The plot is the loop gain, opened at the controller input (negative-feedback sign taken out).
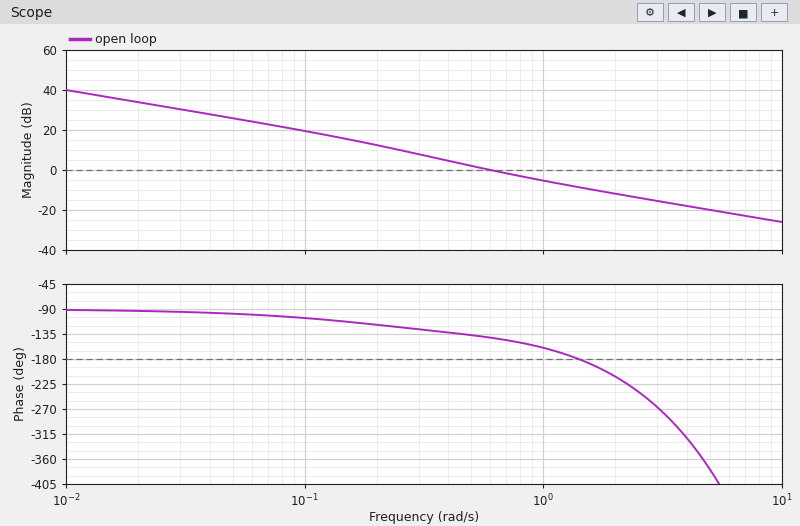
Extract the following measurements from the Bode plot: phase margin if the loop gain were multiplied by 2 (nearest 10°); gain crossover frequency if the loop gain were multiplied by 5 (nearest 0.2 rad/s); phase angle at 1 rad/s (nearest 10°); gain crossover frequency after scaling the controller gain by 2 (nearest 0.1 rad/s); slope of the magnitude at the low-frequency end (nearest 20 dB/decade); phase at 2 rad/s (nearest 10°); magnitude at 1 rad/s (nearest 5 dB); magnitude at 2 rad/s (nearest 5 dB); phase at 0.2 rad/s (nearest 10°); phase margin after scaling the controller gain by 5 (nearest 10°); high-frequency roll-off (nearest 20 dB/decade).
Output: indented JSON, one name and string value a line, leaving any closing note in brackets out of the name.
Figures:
{
  "phase margin if the loop gain were multiplied by 2": "20°",
  "gain crossover frequency if the loop gain were multiplied by 5": "2.6 rad/s",
  "phase angle at 1 rad/s": "-160°",
  "gain crossover frequency after scaling the controller gain by 2": "1.1 rad/s",
  "slope of the magnitude at the low-frequency end": "-20 dB/decade",
  "phase at 2 rad/s": "-210°",
  "magnitude at 1 rad/s": "-5 dB",
  "magnitude at 2 rad/s": "-10 dB",
  "phase at 0.2 rad/s": "-120°",
  "phase margin after scaling the controller gain by 5": "-60°",
  "high-frequency roll-off": "-20 dB/decade"
}
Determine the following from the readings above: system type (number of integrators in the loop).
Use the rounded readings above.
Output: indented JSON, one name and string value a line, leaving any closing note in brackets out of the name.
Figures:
{
  "system type": "1"
}
